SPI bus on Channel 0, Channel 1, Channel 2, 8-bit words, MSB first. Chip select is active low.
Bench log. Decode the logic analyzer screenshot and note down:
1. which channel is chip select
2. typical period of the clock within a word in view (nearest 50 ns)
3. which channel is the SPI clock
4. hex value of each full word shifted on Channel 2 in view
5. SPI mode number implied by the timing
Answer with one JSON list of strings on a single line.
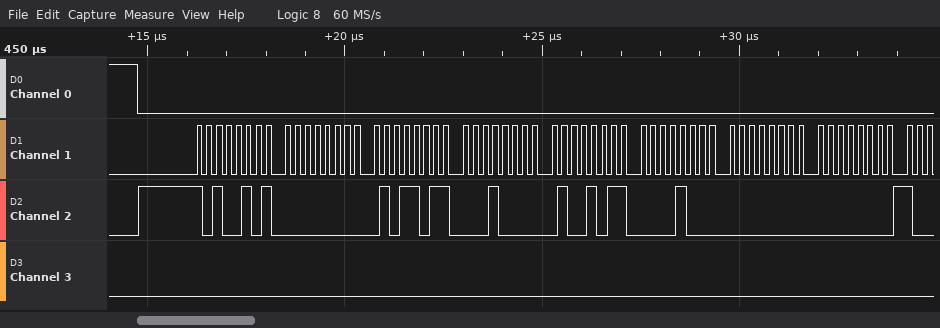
["Channel 0", "250 ns", "Channel 1", "A5, 00, 5B, 10, 4B, 08, 00, 00", "0"]
